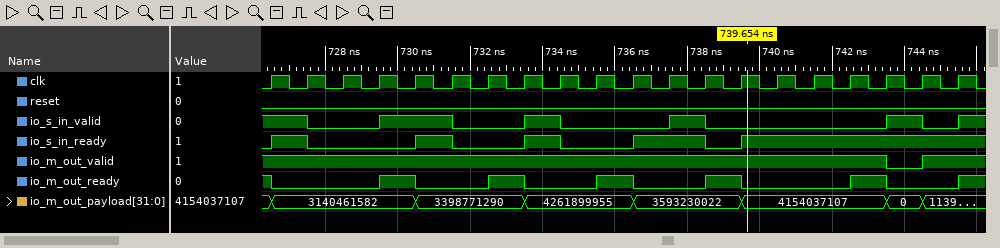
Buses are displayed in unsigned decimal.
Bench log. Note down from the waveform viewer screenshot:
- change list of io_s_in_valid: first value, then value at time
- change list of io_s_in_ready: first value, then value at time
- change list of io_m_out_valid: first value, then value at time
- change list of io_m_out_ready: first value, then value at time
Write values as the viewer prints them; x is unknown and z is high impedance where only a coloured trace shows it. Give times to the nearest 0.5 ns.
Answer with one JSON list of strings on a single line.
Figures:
["1, 0 at 727.5 ns, 1 at 729.5 ns, 0 at 731.5 ns, 1 at 733.5 ns, 0 at 734.5 ns, 1 at 737.5 ns, 0 at 738.5 ns, 1 at 743.5 ns, 0 at 744.5 ns, 1 at 745.5 ns", "0, 1 at 726.5 ns, 0 at 727.5 ns, 1 at 730.5 ns, 0 at 731.5 ns, 1 at 733.5 ns, 0 at 734.5 ns, 1 at 736.5 ns, 0 at 738.5 ns, 1 at 739.5 ns", "1, 0 at 743.5 ns, 1 at 744.5 ns", "1, 0 at 726.5 ns, 1 at 729.5 ns, 0 at 730.5 ns, 1 at 732.5 ns, 0 at 733.5 ns, 1 at 735.5 ns, 0 at 736.5 ns, 1 at 738.5 ns, 0 at 739.5 ns, 1 at 742.5 ns, 0 at 743.5 ns, 1 at 745.5 ns"]
